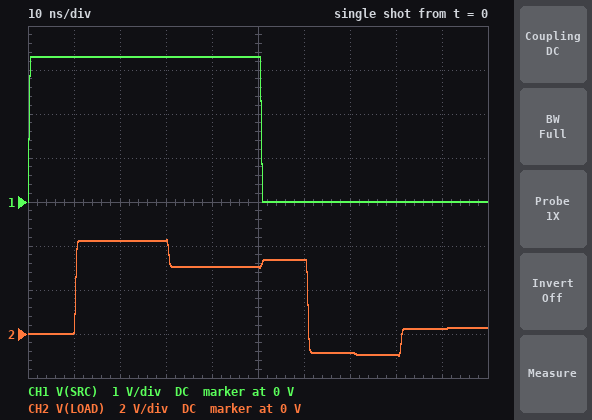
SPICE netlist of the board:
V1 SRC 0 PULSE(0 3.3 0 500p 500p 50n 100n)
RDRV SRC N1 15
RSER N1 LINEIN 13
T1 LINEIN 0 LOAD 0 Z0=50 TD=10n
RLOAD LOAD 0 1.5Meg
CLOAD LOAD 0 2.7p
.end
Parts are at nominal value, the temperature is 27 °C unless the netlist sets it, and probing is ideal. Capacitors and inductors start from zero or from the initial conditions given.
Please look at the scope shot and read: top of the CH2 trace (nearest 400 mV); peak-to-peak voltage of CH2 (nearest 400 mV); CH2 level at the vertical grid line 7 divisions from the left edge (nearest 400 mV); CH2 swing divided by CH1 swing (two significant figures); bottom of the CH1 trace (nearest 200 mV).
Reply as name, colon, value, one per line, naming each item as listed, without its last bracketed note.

top of the CH2 trace: 4.4 V
peak-to-peak voltage of CH2: 5.2 V
CH2 level at the vertical grid line 7 divisions from the left edge: -800 mV
CH2 swing divided by CH1 swing: 1.6
bottom of the CH1 trace: 0 V
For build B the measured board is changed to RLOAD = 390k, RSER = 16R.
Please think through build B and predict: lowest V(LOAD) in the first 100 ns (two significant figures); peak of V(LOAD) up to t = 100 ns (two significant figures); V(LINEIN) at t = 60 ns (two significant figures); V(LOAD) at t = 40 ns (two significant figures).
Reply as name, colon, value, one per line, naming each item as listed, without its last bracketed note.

lowest V(LOAD) in the first 100 ns: -830 mV
peak of V(LOAD) up to t = 100 ns: 4.1 V
V(LINEIN) at t = 60 ns: 1.2 V
V(LOAD) at t = 40 ns: 3.1 V
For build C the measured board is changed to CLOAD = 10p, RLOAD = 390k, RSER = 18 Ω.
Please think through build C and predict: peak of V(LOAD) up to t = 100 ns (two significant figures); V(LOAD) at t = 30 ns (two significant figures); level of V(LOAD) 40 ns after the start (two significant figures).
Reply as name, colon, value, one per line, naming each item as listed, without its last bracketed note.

peak of V(LOAD) up to t = 100 ns: 4.1 V
V(LOAD) at t = 30 ns: 4.0 V
level of V(LOAD) 40 ns after the start: 3.2 V
